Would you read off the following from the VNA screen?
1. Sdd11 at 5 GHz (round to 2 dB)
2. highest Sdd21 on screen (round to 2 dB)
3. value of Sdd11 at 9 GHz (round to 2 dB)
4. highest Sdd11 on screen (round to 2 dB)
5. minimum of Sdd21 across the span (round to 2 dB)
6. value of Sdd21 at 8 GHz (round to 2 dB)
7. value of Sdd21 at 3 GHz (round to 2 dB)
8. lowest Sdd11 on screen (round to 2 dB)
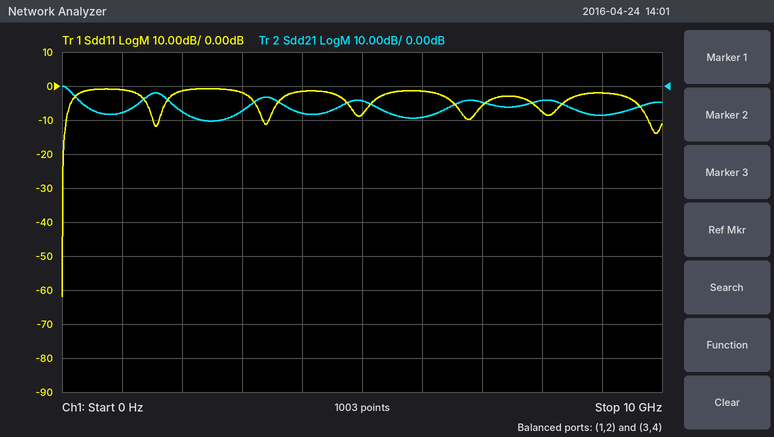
-8 dB
0 dB
-2 dB
0 dB
-10 dB
-4 dB
-8 dB
-62 dB
